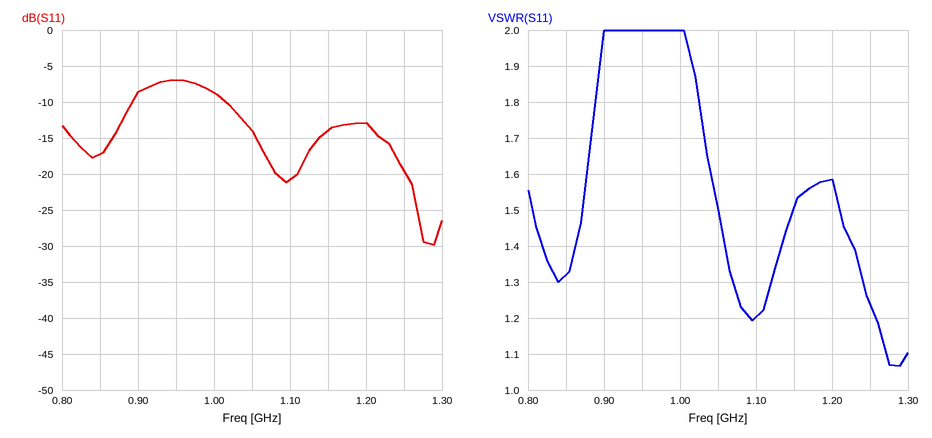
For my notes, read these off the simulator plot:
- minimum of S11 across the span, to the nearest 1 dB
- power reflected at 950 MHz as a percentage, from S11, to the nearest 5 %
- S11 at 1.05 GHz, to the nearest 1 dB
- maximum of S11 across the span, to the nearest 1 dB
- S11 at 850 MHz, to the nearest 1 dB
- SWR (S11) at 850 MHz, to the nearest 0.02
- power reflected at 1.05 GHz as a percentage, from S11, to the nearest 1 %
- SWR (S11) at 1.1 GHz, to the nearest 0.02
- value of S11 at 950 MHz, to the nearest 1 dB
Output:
-30 dB
20 %
-14 dB
-7 dB
-17 dB
1.32
4 %
1.20
-7 dB
